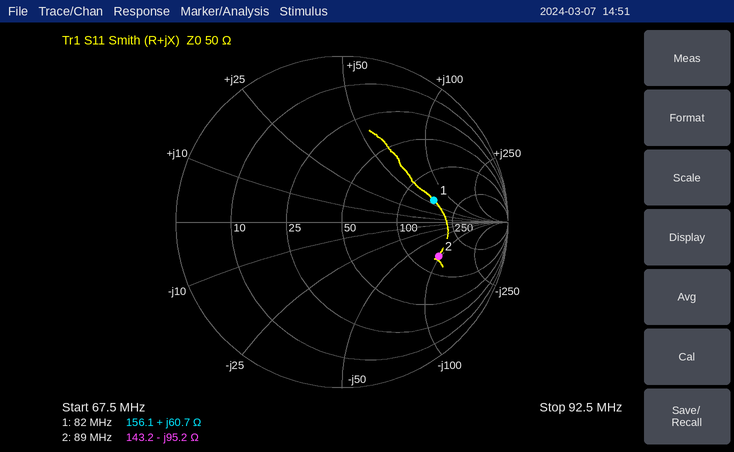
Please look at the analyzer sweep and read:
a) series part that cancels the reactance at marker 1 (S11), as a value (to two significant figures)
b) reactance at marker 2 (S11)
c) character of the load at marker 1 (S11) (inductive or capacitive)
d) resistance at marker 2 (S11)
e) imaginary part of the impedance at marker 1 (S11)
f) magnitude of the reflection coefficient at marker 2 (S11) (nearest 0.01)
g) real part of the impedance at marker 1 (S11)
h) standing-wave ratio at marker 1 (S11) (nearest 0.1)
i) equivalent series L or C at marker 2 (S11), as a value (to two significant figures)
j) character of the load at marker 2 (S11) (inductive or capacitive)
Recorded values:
32 pF
-95.2 Ω
inductive
143.2 Ω
+60.7 Ω
0.62
156.1 Ω
3.6
19 pF
capacitive
